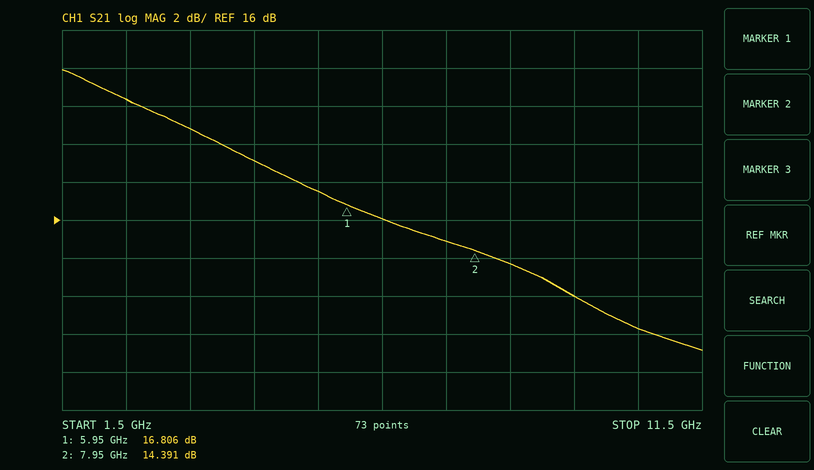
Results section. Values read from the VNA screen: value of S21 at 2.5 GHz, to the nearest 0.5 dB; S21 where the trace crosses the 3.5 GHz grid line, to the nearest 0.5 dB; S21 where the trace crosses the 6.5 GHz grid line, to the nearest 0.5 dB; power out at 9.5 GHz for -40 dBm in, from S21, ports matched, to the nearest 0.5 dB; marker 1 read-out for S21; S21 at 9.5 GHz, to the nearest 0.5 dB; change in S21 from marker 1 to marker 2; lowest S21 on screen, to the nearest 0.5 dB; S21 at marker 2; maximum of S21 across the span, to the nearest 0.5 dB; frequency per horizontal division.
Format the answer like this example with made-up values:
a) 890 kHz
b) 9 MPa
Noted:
a) 22.5 dB
b) 21.0 dB
c) 16.0 dB
d) -28.0 dBm
e) 16.806 dB
f) 12.0 dB
g) -2.415 dB
h) 9.0 dB
i) 14.391 dB
j) 24.0 dB
k) 1 GHz
